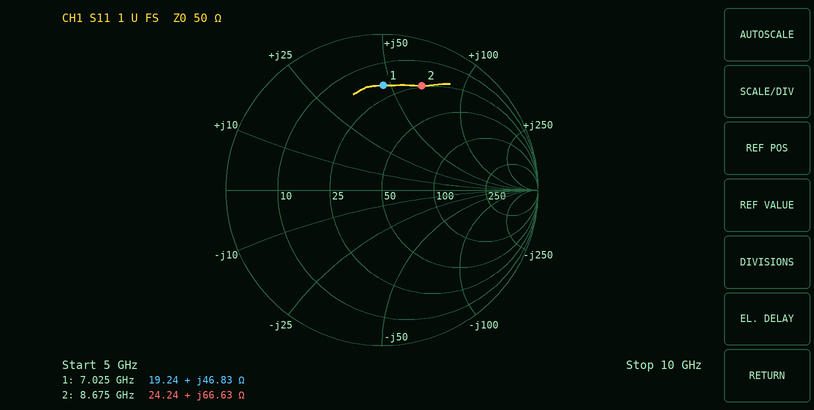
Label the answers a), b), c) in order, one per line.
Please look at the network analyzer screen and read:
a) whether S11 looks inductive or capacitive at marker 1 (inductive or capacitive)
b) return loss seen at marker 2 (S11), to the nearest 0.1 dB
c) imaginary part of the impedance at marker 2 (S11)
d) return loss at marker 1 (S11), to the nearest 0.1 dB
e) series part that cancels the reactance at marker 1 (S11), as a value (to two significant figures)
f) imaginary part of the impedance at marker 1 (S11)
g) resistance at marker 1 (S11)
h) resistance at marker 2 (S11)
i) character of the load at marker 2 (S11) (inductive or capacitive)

a) inductive
b) 2.9 dB
c) +66.63 Ω
d) 3.5 dB
e) 480 fF
f) +46.83 Ω
g) 19.24 Ω
h) 24.24 Ω
i) inductive
